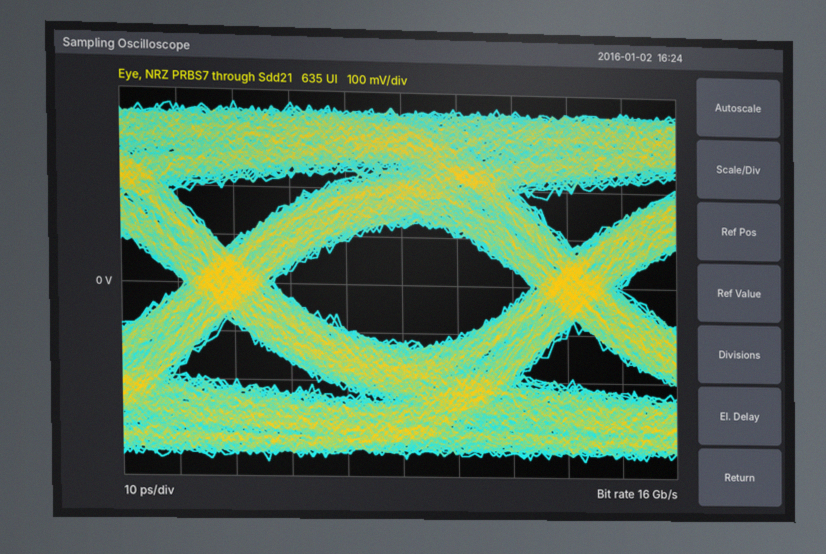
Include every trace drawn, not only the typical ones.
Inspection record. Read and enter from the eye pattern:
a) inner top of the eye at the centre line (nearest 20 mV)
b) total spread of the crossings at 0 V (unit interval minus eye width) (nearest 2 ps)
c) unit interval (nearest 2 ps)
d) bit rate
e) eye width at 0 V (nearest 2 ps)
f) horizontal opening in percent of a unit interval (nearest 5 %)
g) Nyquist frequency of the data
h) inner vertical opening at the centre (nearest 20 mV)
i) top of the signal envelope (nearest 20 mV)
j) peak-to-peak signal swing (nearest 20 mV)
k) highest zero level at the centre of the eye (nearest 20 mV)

120 mV
16 ps
62 ps
16 Gb/s
46 ps
75 %
8 GHz
240 mV
380 mV
740 mV
-120 mV
